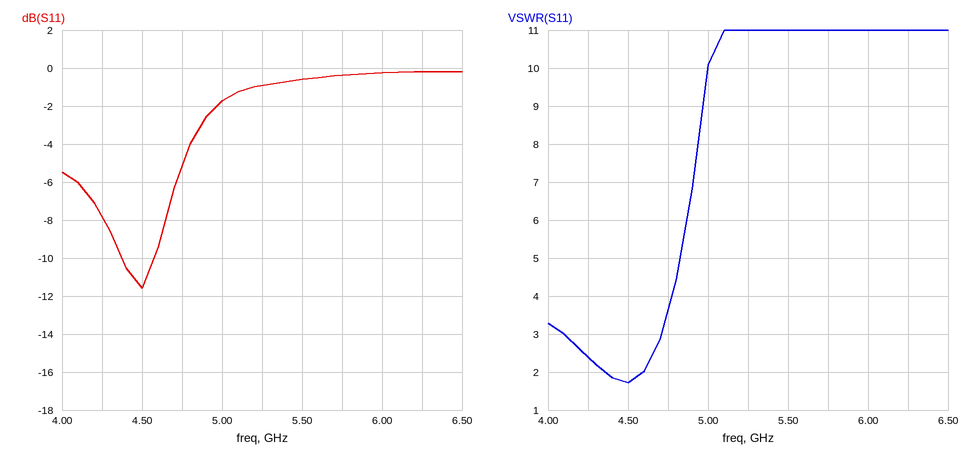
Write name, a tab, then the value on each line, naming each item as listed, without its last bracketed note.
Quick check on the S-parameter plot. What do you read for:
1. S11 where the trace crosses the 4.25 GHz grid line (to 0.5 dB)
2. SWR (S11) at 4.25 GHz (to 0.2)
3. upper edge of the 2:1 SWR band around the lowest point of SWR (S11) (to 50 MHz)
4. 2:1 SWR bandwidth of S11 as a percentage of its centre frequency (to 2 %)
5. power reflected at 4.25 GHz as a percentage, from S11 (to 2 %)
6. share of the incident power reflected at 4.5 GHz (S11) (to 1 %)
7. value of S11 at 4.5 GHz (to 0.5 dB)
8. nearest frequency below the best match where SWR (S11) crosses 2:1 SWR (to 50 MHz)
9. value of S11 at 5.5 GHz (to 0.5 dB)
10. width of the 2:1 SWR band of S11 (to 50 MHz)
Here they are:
S11 where the trace crosses the 4.25 GHz grid line	-8.0 dB
SWR (S11) at 4.25 GHz	2.4
upper edge of the 2:1 SWR band around the lowest point of SWR (S11)	4.60 GHz
2:1 SWR bandwidth of S11 as a percentage of its centre frequency	6 %
power reflected at 4.25 GHz as a percentage, from S11	16 %
share of the incident power reflected at 4.5 GHz (S11)	7 %
value of S11 at 4.5 GHz	-11.5 dB
nearest frequency below the best match where SWR (S11) crosses 2:1 SWR	4.35 GHz
value of S11 at 5.5 GHz	-0.5 dB
width of the 2:1 SWR band of S11	250 MHz
